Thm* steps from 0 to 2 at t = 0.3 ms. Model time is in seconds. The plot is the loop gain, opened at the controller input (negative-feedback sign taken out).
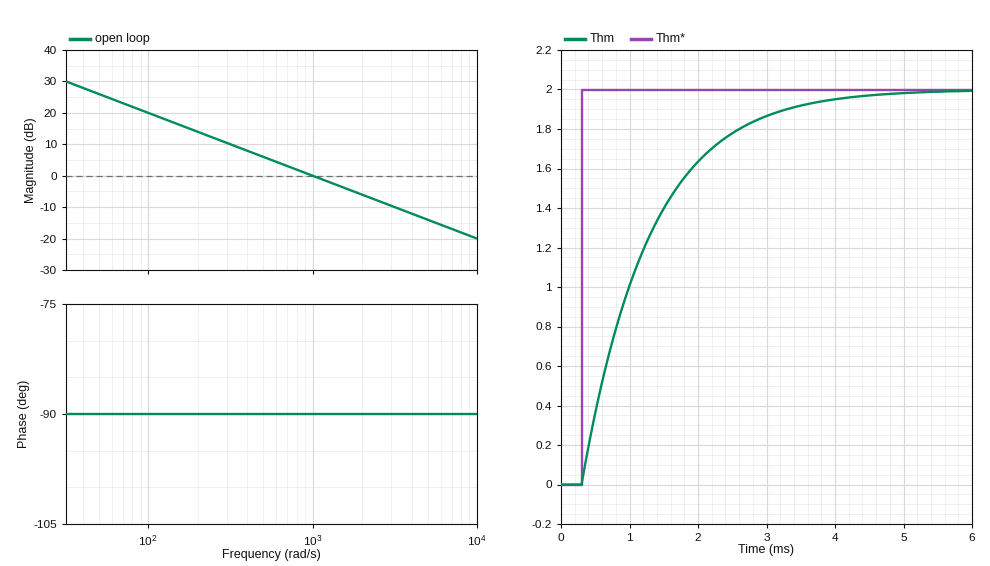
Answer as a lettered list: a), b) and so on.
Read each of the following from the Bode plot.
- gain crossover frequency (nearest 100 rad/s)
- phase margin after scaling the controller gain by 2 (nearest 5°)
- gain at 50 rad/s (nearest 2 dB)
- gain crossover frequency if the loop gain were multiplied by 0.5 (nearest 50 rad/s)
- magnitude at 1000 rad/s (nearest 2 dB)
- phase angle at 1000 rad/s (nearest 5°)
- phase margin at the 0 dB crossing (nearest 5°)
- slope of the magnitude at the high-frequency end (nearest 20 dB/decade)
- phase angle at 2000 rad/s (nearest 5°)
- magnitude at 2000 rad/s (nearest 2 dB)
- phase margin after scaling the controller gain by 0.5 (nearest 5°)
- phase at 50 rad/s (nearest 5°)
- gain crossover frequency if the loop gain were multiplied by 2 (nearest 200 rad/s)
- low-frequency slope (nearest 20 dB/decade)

a) 1000 rad/s
b) 90°
c) 26 dB
d) 500 rad/s
e) 0 dB
f) -90°
g) 90°
h) -20 dB/decade
i) -90°
j) -6 dB
k) 90°
l) -90°
m) 2000 rad/s
n) -20 dB/decade
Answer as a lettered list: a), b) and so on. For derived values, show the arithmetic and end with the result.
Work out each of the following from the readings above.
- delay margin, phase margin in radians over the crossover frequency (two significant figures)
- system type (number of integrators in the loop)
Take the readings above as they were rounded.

a) 90 × π / 180 / 1000 = 0.0016 s
b) 1
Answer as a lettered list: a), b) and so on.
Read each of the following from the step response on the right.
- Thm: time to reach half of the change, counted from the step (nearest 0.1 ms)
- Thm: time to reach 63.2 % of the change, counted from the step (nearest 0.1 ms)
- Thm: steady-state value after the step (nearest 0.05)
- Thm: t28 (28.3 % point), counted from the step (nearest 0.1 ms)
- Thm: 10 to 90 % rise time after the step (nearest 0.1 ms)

a) 0.7 ms
b) 1.0 ms
c) 2.00
d) 0.3 ms
e) 2.2 ms
